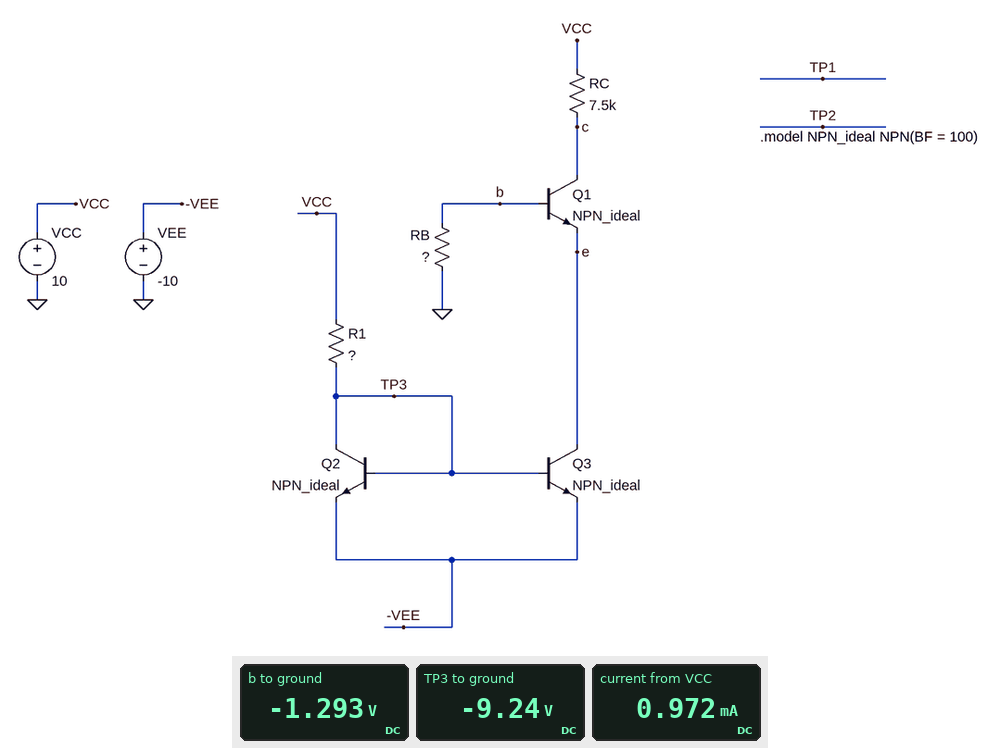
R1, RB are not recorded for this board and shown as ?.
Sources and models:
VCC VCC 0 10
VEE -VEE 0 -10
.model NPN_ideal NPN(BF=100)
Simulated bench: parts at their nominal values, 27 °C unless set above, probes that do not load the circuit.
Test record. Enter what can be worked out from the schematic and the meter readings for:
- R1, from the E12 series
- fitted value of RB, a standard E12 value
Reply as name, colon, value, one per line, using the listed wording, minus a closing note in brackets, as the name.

R1, from the E12 series: 39 kΩ
fitted value of RB, a standard E12 value: 270 kΩ
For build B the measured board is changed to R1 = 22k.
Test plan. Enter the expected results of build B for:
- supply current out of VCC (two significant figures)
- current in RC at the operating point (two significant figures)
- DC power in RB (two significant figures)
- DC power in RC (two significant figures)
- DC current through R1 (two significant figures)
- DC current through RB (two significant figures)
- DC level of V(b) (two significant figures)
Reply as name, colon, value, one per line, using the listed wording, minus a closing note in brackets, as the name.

supply current out of VCC: 1.7 mA
current in RC at the operating point: 850 µA
DC power in RB: 19 µW
DC power in RC: 5.4 mW
DC current through R1: 870 µA
DC current through RB: 8.5 µA
DC level of V(b): -2.3 V
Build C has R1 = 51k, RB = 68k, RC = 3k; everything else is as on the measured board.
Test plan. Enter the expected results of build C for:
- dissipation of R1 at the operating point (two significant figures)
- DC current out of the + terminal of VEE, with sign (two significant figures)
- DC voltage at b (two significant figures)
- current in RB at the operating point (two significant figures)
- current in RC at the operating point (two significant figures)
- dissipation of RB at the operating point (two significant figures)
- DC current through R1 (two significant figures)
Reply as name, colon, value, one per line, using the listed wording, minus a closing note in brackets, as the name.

dissipation of R1 at the operating point: 7.3 mW
DC current out of the + terminal of VEE, with sign: -750 µA
DC voltage at b: -250 mV
current in RB at the operating point: 3.7 µA
current in RC at the operating point: 370 µA
dissipation of RB at the operating point: 910 nW
DC current through R1: 380 µA
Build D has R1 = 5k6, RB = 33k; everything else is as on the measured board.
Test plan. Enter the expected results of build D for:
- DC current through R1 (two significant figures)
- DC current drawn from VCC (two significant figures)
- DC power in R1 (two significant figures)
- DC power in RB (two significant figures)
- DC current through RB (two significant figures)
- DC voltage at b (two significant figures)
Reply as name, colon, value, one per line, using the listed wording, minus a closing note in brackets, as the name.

DC current through R1: 3.4 mA
DC current drawn from VCC: 6.1 mA
DC power in R1: 66 mW
DC power in RB: 2.5 mW
DC current through RB: 280 µA
DC voltage at b: -9.1 V
